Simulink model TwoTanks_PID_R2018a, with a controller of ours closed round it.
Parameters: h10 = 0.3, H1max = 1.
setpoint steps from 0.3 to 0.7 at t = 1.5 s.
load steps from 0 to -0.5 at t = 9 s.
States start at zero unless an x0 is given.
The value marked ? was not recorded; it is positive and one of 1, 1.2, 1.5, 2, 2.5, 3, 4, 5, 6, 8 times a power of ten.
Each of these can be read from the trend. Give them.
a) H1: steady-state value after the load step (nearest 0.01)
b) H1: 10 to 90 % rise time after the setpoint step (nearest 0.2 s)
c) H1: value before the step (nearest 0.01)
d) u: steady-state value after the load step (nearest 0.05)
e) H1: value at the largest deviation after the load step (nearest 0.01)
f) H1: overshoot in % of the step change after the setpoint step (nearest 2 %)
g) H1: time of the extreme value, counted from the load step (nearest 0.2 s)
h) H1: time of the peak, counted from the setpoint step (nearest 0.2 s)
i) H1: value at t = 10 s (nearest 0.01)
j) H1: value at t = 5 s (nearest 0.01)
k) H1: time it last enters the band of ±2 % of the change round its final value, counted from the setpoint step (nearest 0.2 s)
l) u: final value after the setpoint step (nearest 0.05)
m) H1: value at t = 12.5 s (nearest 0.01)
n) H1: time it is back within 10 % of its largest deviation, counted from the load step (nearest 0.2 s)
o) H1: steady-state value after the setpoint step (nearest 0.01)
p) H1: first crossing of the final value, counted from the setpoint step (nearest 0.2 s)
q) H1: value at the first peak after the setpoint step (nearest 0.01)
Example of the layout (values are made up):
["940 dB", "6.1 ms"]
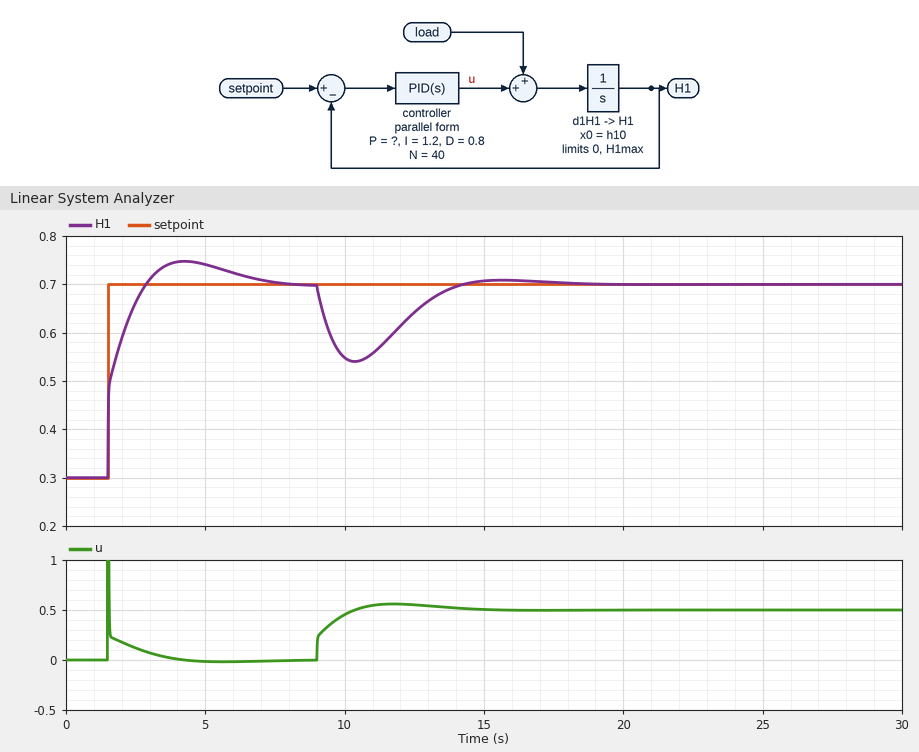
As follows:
["0.70", "1.0 s", "0.30", "0.50", "0.54", "12 %", "1.4 s", "2.8 s", "0.55", "0.74", "5.6 s", "0.00", "0.64", "4.6 s", "0.70", "1.4 s", "0.75"]
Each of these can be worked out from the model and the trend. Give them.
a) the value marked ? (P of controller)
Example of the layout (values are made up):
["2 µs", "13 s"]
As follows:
["2"]
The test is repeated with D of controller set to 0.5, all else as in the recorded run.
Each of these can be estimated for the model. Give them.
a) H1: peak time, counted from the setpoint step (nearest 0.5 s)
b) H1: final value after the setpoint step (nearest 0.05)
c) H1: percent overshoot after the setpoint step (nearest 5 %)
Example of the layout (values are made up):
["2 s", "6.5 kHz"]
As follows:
["2.5 s", "0.70", "15 %"]
